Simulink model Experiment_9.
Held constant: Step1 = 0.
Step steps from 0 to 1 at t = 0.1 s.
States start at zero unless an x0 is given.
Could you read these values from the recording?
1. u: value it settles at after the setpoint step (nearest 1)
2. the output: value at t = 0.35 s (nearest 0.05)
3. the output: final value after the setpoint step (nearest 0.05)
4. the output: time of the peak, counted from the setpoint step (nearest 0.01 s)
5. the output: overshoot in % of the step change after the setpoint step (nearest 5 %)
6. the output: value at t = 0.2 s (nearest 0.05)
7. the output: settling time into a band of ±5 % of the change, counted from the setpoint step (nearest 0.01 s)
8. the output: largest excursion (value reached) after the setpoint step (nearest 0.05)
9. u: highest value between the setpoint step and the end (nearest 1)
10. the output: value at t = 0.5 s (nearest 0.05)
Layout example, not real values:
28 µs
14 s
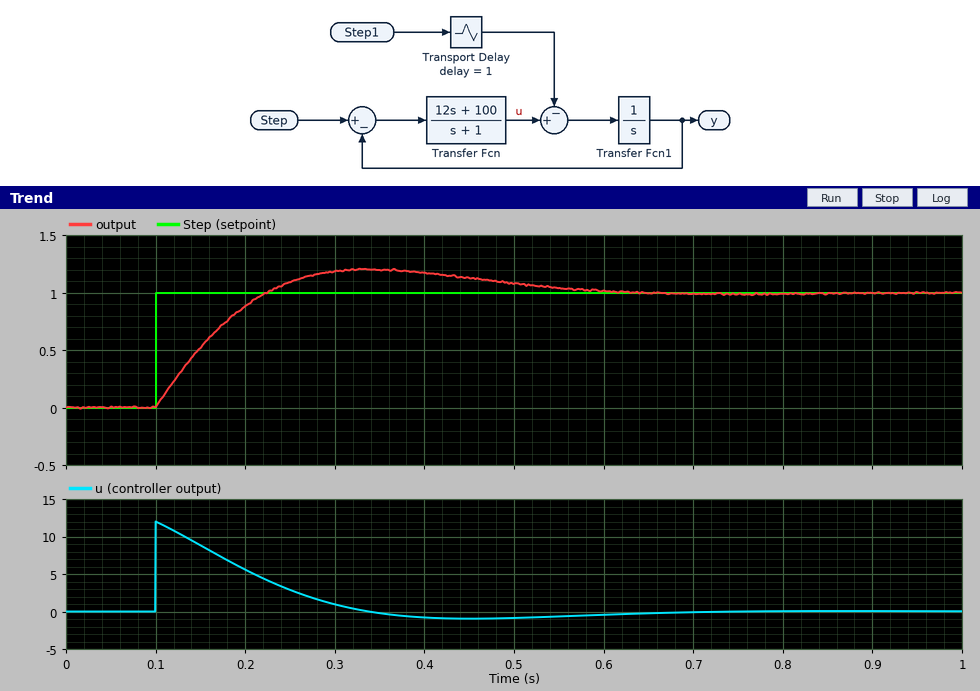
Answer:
0
1.20
1.00
0.24 s
20 %
0.90
0.44 s
1.20
12
1.10
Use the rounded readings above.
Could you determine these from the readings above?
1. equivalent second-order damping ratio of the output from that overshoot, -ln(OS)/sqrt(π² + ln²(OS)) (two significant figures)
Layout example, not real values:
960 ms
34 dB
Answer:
0.46
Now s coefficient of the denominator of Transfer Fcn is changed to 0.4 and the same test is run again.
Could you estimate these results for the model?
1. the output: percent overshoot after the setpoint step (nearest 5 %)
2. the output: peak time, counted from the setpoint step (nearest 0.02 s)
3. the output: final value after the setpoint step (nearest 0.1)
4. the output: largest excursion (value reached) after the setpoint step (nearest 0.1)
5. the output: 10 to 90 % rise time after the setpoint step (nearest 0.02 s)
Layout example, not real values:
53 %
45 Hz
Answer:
10 %
0.14 s
1.0
1.1
0.06 s
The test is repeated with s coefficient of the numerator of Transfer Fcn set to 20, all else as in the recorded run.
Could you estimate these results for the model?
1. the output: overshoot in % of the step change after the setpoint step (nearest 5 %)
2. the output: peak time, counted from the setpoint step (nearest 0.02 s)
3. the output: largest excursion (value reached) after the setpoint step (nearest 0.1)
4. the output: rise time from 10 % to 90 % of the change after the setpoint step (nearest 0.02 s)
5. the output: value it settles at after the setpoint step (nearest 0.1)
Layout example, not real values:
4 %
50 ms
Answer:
10 %
0.20 s
1.1
0.08 s
1.0
